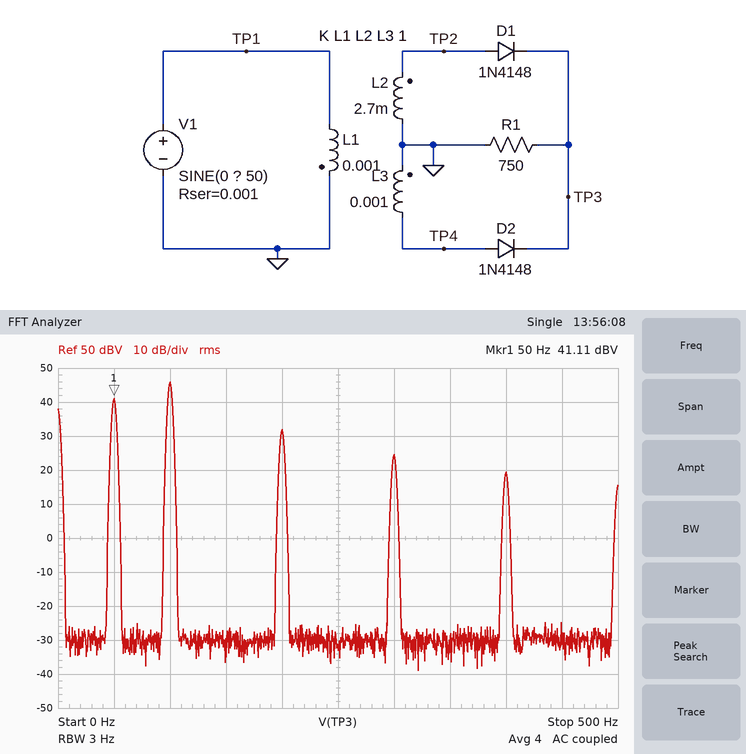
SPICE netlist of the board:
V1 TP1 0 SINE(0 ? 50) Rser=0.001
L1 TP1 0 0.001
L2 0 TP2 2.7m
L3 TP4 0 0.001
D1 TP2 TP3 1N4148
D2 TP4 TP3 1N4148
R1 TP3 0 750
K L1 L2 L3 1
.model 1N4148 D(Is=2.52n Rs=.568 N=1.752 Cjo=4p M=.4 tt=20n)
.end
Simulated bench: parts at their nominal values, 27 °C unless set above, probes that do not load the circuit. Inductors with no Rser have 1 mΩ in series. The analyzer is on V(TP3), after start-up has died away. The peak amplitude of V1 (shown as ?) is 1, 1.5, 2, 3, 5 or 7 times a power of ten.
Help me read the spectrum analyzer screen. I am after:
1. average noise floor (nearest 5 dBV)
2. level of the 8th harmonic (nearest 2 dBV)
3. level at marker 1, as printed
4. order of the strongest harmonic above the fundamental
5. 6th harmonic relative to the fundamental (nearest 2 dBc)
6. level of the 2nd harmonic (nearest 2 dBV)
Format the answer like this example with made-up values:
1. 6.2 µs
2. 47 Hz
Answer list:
1. -30 dBV
2. 20 dBV
3. 41.11 dBV
4. 2
5. -16 dBc
6. 46 dBV
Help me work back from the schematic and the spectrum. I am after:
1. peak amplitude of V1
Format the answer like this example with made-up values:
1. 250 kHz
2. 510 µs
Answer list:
1. 500 V
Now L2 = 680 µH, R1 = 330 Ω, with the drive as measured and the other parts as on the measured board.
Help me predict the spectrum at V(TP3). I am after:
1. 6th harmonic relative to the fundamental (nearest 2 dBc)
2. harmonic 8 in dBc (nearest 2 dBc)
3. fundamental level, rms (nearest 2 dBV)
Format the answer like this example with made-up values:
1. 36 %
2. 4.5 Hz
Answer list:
1. -8 dBc
2. -14 dBc
3. 30 dBV
